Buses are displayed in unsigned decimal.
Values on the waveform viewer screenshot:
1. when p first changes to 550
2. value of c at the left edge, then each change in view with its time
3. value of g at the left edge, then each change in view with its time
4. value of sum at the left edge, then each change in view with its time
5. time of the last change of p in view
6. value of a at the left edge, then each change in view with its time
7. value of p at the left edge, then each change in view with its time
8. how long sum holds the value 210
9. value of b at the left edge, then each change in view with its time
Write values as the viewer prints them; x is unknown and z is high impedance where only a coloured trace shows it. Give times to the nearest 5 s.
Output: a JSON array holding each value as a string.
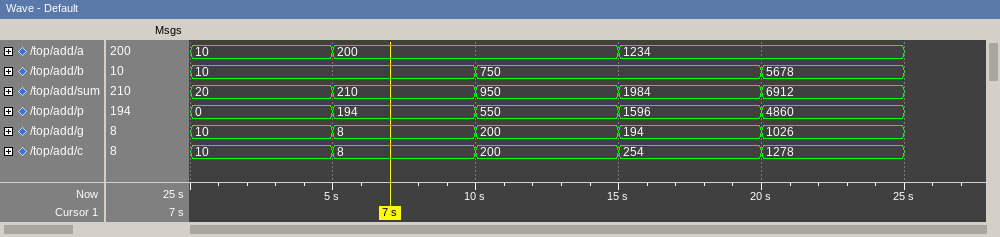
["10 s", "10, 8 at 5 s, 200 at 10 s, 254 at 15 s, 1278 at 20 s", "10, 8 at 5 s, 200 at 10 s, 194 at 15 s, 1026 at 20 s", "20, 210 at 5 s, 950 at 10 s, 1984 at 15 s, 6912 at 20 s", "20 s", "10, 200 at 5 s, 1234 at 15 s", "0, 194 at 5 s, 550 at 10 s, 1596 at 15 s, 4860 at 20 s", "5 s", "10, 750 at 10 s, 5678 at 20 s"]
